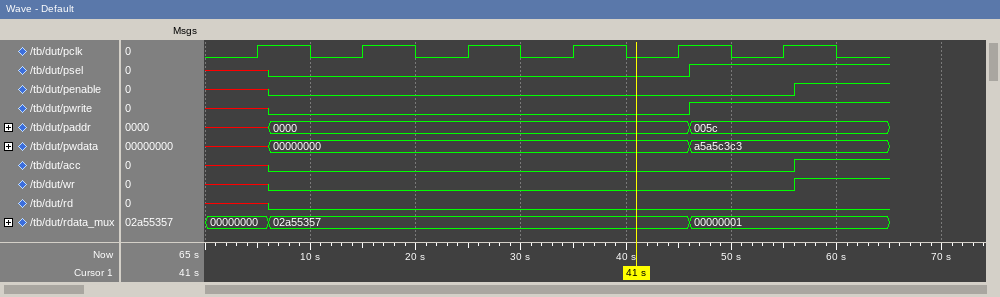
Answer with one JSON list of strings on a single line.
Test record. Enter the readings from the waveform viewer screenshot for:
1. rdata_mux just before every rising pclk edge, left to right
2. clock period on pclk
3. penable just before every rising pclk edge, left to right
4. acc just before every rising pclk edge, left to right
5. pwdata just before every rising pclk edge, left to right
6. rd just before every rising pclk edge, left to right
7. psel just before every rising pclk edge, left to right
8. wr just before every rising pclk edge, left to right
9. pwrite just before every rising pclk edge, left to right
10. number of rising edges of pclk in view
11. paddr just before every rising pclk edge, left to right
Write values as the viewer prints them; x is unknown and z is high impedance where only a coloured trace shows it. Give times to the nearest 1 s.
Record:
["00000000, 02a55357, 02a55357, 02a55357, 02a55357, 00000001", "10 s", "x 0 0 0 0 0", "x 0 0 0 0 0", "x, 00000000, 00000000, 00000000, 00000000, a5a5c3c3", "x 0 0 0 0 0", "x 0 0 0 0 1", "x 0 0 0 0 0", "x 0 0 0 0 1", "6", "x, 0000, 0000, 0000, 0000, 005c"]
